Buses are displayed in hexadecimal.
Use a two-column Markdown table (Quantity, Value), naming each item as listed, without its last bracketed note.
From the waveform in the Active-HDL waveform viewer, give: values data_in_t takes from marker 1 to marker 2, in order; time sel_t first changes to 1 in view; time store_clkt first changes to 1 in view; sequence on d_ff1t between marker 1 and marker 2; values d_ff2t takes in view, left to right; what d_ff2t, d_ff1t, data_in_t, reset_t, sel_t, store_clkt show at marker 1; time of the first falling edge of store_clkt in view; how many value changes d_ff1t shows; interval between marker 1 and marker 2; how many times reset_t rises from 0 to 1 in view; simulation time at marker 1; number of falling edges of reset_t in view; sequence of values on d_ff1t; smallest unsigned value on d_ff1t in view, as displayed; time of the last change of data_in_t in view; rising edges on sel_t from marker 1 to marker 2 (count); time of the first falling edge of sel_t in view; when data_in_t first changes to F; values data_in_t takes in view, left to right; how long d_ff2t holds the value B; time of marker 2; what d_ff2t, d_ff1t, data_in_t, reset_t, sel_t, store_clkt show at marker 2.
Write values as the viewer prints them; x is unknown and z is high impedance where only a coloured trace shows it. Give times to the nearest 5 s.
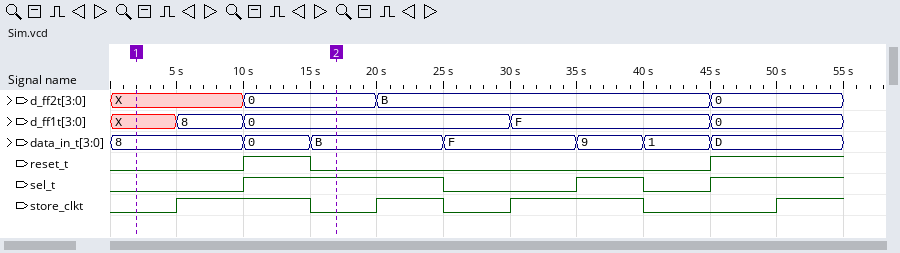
| Quantity | Value |
|---|---|
| values data_in_t takes from marker 1 to marker 2, in order | 8, 0, B |
| time sel_t first changes to 1 in view | 10 s |
| time store_clkt first changes to 1 in view | 5 s |
| sequence on d_ff1t between marker 1 and marker 2 | X, 8, 0 |
| values d_ff2t takes in view, left to right | X, 0, B, 0 |
| what d_ff2t, d_ff1t, data_in_t, reset_t, sel_t, store_clkt show at marker 1 | d_ff2t=X, d_ff1t=X, data_in_t=8, reset_t=0, sel_t=0, store_clkt=0 |
| time of the first falling edge of store_clkt in view | 15 s |
| how many value changes d_ff1t shows | 4 |
| interval between marker 1 and marker 2 | 15 s |
| how many times reset_t rises from 0 to 1 in view | 2 |
| simulation time at marker 1 | 0 s |
| number of falling edges of reset_t in view | 1 |
| sequence of values on d_ff1t | X, 8, 0, F, 0 |
| smallest unsigned value on d_ff1t in view, as displayed | 0 |
| time of the last change of data_in_t in view | 45 s |
| rising edges on sel_t from marker 1 to marker 2 | 1 |
| time of the first falling edge of sel_t in view | 25 s |
| when data_in_t first changes to F | 25 s |
| values data_in_t takes in view, left to right | 8, 0, B, F, 9, 1, D |
| how long d_ff2t holds the value B | 25 s |
| time of marker 2 | 15 s |
| what d_ff2t, d_ff1t, data_in_t, reset_t, sel_t, store_clkt show at marker 2 | d_ff2t=0, d_ff1t=0, data_in_t=B, reset_t=0, sel_t=1, store_clkt=0 |
